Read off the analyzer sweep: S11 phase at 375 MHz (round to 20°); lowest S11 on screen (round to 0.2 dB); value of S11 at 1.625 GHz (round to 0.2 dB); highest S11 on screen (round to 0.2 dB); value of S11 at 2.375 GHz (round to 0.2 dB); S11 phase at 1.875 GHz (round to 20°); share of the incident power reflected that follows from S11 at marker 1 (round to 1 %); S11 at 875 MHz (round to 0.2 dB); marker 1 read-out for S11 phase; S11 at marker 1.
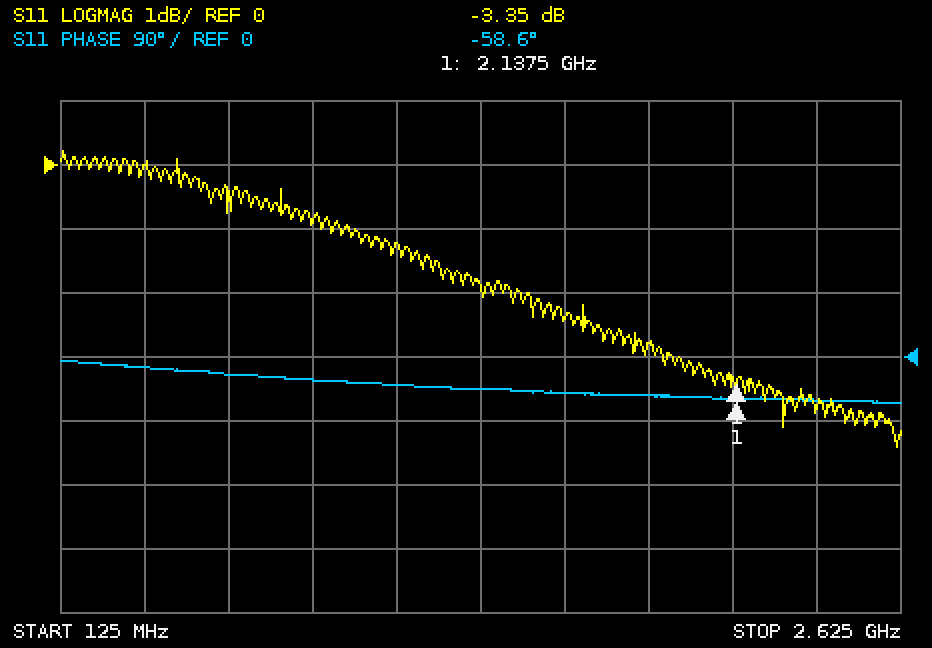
-20°
-4.4 dB
-2.4 dB
0.2 dB
-3.8 dB
-60°
46 %
-0.8 dB
-58.6°
-3.35 dB
